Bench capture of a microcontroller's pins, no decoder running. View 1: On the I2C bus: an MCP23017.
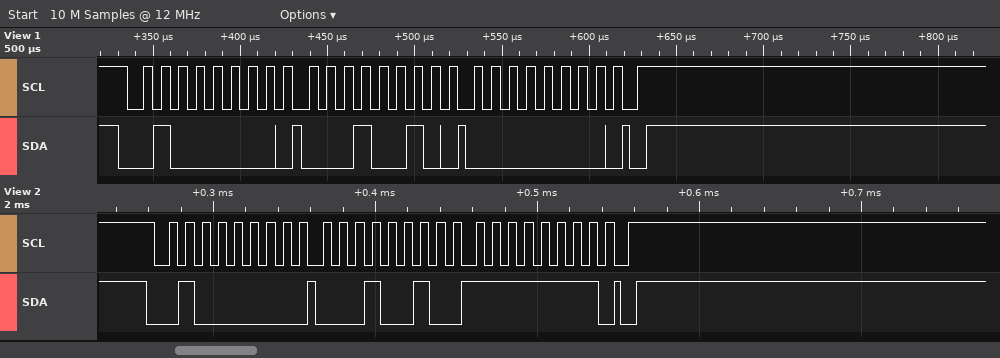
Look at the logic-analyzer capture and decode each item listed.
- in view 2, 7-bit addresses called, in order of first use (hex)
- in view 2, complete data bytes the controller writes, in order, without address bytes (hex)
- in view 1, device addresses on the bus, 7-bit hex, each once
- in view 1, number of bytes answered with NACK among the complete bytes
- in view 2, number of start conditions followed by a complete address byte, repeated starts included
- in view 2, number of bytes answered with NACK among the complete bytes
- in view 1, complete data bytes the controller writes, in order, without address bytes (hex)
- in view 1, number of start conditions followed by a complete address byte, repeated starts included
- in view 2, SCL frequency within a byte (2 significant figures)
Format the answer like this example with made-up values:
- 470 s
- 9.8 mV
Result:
- 0x20
- 12 FF
- 0x20
- 0
- 1
- 0
- 12 00
- 1
- 100 kHz
